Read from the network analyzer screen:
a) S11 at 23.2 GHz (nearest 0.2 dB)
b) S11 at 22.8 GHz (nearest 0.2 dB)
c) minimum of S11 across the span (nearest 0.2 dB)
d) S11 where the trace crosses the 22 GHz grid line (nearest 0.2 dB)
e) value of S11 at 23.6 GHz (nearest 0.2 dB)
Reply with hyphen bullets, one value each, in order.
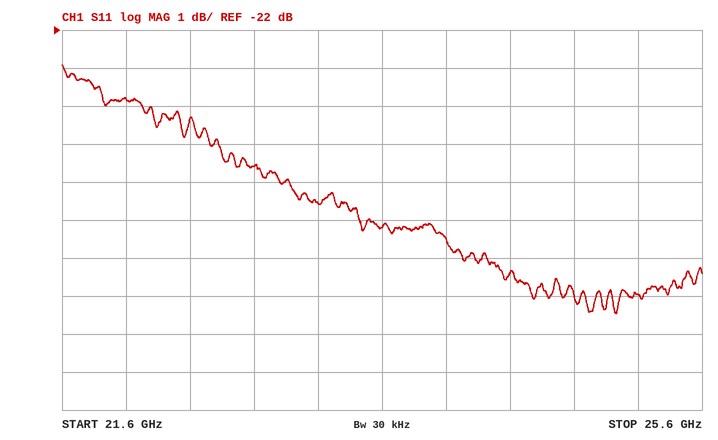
- -26.6 dB
- -25.6 dB
- -29.4 dB
- -23.8 dB
- -27.2 dB
